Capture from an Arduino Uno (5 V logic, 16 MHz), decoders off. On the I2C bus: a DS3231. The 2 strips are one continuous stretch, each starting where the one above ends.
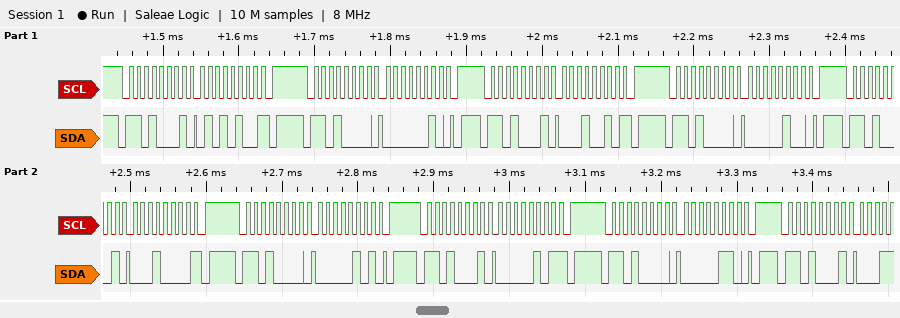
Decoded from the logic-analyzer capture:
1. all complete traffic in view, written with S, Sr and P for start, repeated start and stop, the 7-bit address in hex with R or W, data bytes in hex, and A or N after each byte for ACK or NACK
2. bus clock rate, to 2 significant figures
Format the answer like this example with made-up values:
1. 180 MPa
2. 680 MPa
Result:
1. S 68R A 54 N P S 68W A 02 A P S 68R A 12 N P S 68W A 04 A P S 68R A 10 N P S 68W A 05 A P S 68R A 05 N P S 68W A 06 A P S 68R A
2. 100 kHz
